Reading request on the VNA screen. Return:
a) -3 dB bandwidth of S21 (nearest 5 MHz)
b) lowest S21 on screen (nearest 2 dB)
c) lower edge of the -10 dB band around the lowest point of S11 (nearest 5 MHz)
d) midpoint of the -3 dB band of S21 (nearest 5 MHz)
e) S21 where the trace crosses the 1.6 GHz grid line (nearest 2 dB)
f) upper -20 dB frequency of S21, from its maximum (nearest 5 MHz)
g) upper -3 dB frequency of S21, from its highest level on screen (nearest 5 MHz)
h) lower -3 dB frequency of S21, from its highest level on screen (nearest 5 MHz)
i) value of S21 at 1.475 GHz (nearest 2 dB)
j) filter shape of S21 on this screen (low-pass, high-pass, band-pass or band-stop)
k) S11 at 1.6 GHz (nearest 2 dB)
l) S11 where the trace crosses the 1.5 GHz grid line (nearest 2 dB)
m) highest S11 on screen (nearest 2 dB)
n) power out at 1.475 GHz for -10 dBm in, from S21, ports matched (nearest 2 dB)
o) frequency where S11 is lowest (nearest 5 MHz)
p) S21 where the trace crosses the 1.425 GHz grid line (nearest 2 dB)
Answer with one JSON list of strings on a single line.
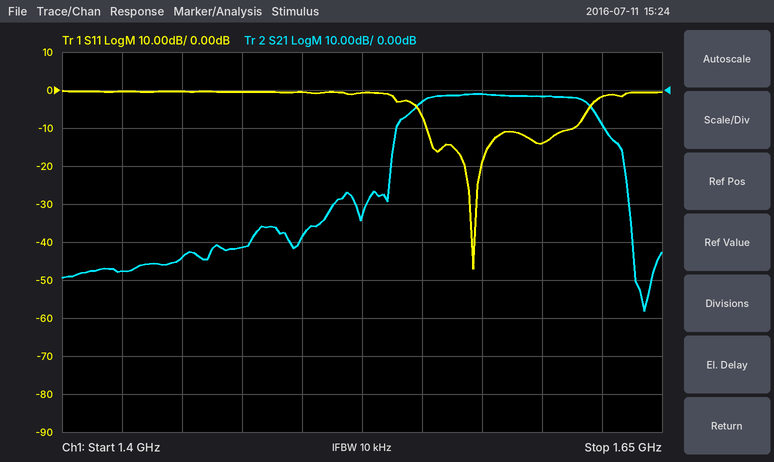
["70 MHz", "-58 dB", "1.550 GHz", "1.585 GHz", "-2 dB", "1.635 GHz", "1.620 GHz", "1.550 GHz", "-42 dB", "band-pass", "-14 dB", "0 dB", "0 dB", "-52 dBm", "1.570 GHz", "-48 dB"]
